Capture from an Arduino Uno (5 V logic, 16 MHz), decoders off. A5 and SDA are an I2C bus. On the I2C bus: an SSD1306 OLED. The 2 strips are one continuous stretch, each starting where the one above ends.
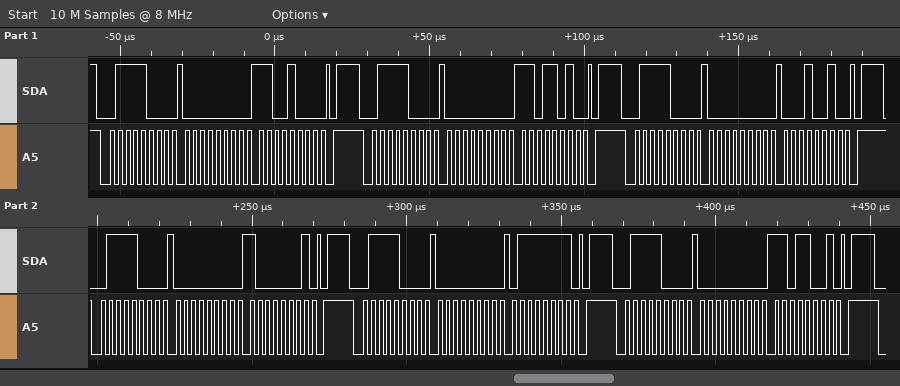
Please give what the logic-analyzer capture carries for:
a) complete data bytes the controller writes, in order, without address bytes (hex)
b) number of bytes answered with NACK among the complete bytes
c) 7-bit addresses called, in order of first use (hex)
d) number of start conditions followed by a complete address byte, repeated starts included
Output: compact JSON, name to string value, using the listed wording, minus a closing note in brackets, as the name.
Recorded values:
{"complete data bytes the controller writes, in order, without address bytes": "00 C8 00 DA 00 12 00 81 00 7F 00 D9", "number of bytes answered with NACK among the complete bytes": "0", "7-bit addresses called, in order of first use": "0x3C", "number of start conditions followed by a complete address byte, repeated starts included": "6"}
